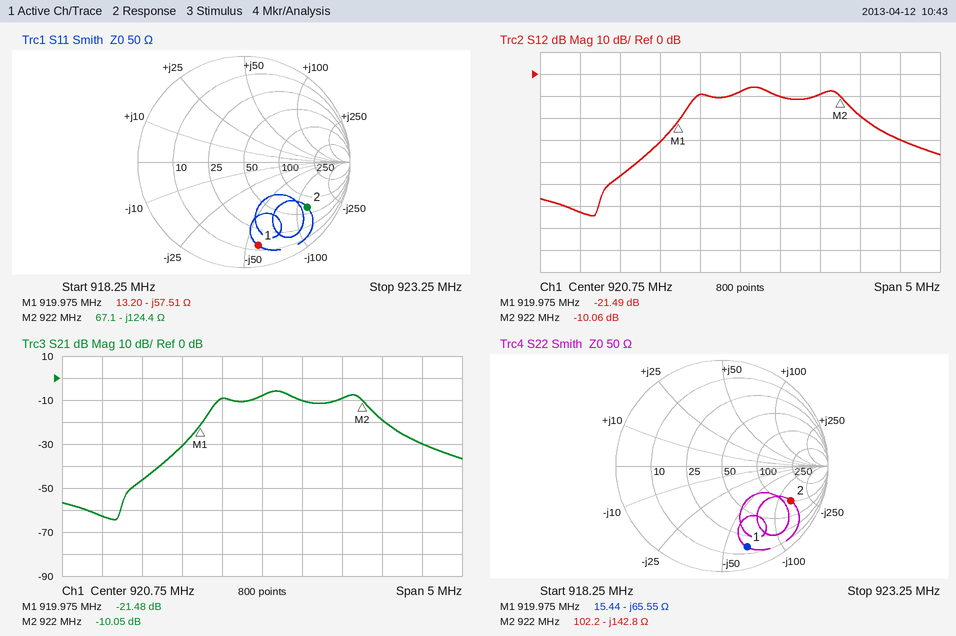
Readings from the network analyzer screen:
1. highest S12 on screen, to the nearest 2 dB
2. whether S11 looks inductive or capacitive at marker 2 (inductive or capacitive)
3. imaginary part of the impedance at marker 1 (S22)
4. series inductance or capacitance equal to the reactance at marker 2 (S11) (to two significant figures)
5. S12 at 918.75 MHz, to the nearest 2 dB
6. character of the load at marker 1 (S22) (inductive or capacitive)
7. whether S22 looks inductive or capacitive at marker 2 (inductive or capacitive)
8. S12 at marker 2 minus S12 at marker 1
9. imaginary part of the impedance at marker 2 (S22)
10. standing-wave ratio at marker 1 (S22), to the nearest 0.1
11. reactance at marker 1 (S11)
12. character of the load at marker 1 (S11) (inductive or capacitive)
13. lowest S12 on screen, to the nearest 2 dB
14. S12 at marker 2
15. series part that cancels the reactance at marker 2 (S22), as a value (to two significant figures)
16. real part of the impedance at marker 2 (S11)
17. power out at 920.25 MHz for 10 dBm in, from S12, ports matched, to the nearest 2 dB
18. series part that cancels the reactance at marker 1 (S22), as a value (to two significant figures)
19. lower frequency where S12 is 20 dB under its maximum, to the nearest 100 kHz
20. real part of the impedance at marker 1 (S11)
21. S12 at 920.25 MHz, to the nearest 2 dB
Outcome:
-6 dB
capacitive
-65.55 Ω
1.4 pF
-62 dB
capacitive
capacitive
11.43 dB
-142.8 Ω
9.0
-57.51 Ω
capacitive
-64 dB
-10.06 dB
25 nH
67.1 Ω
0 dBm
11 nH
919.9 MHz
13.20 Ω
-10 dB
